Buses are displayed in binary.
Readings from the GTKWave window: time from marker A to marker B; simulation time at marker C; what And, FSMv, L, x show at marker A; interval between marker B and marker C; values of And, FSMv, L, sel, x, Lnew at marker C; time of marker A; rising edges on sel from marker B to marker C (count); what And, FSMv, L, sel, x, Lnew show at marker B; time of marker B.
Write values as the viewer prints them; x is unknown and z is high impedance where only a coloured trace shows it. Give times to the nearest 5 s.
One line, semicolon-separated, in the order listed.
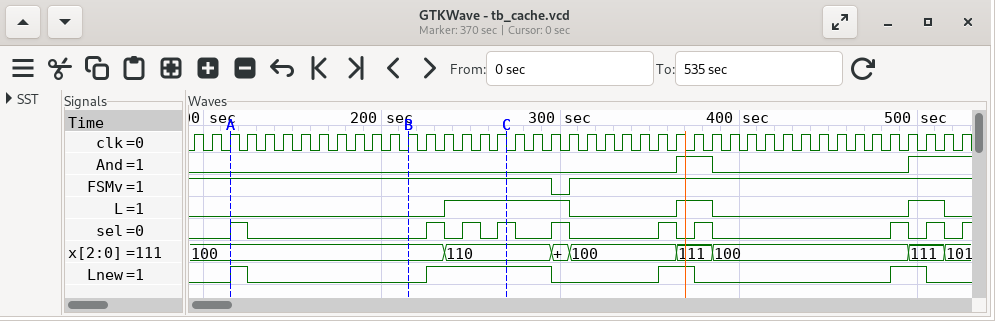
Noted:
100 s; 270 s; And=0, FSMv=1, L=0, x=100; 55 s; And=0, FSMv=1, L=1, sel=1, x=110, Lnew=1; 115 s; 3; And=0, FSMv=1, L=0, sel=0, x=100, Lnew=0; 215 s
